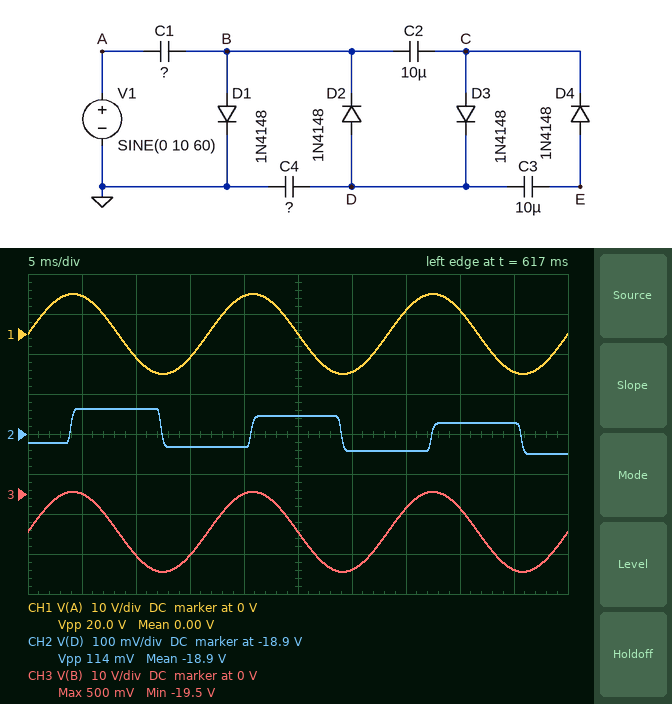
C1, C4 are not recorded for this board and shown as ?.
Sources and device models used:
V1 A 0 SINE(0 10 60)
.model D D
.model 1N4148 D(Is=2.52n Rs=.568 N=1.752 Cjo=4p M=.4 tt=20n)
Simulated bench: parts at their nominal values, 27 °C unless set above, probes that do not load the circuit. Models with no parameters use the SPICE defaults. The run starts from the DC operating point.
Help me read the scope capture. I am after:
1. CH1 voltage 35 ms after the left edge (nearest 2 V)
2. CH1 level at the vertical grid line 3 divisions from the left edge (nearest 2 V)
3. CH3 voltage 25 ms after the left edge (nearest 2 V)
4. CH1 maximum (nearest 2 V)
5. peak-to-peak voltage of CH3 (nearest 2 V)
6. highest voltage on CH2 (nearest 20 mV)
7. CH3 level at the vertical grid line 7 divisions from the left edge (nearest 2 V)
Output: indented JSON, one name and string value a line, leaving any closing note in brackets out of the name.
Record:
{
  "CH1 voltage 35 ms after the left edge": "6 V",
  "CH1 level at the vertical grid line 3 divisions from the left edge": "-6 V",
  "CH3 voltage 25 ms after the left edge": "-10 V",
  "CH1 maximum": "10 V",
  "peak-to-peak voltage of CH3": "20 V",
  "highest voltage on CH2": "-18.84 V",
  "CH3 level at the vertical grid line 7 divisions from the left edge": "-4 V"
}
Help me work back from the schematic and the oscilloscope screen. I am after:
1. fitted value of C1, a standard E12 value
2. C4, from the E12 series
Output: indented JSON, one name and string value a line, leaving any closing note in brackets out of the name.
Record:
{
  "fitted value of C1, a standard E12 value": "12 µF",
  "C4, from the E12 series": "4.7 µF"
}
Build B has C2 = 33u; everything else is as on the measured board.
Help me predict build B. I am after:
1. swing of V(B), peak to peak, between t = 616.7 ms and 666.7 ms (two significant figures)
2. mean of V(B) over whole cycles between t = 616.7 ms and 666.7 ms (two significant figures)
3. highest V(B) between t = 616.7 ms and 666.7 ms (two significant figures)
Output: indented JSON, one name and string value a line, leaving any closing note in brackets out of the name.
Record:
{
  "swing of V(B), peak to peak, between t = 616.7 ms and 666.7 ms": "20 V",
  "mean of V(B) over whole cycles between t = 616.7 ms and 666.7 ms": "-9.3 V",
  "highest V(B) between t = 616.7 ms and 666.7 ms": "580 mV"
}
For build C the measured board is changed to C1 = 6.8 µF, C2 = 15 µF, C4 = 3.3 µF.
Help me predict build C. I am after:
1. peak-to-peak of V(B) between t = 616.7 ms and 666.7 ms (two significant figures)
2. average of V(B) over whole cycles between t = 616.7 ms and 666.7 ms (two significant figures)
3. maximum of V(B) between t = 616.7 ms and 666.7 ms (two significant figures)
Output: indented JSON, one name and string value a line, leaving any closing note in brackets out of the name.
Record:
{
  "peak-to-peak of V(B) between t = 616.7 ms and 666.7 ms": "20 V",
  "average of V(B) over whole cycles between t = 616.7 ms and 666.7 ms": "-9.3 V",
  "maximum of V(B) between t = 616.7 ms and 666.7 ms": "560 mV"
}
